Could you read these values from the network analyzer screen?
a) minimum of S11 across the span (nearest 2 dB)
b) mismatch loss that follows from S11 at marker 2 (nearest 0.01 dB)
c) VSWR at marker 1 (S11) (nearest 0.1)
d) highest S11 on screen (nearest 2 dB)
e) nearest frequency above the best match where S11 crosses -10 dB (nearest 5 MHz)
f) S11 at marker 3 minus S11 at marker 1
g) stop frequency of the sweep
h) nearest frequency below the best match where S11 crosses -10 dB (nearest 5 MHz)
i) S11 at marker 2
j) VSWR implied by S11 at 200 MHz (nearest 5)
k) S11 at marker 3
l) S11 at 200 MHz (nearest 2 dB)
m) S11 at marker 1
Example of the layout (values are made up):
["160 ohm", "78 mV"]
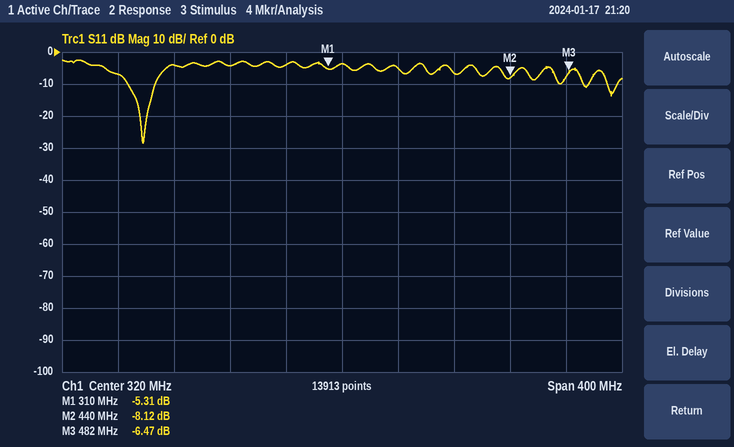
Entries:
["-28 dB", "0.73 dB", "3.4", "-2 dB", "185 MHz", "-1.16 dB", "520 MHz", "165 MHz", "-8.12 dB", "5", "-6.47 dB", "-4 dB", "-5.31 dB"]
